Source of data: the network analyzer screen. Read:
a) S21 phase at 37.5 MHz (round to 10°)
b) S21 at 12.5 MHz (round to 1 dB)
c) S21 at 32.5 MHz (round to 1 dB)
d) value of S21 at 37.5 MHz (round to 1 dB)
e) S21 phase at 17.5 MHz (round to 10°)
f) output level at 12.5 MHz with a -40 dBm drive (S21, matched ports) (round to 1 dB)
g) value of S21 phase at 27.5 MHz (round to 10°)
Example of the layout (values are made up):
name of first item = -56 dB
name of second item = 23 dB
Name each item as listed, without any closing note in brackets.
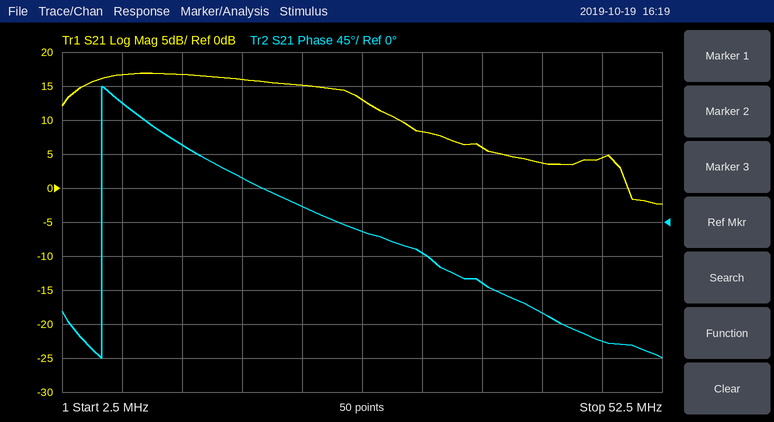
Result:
S21 phase at 37.5 MHz = -80°
S21 at 12.5 MHz = 17 dB
S21 at 32.5 MHz = 8 dB
value of S21 at 37.5 MHz = 6 dB
S21 phase at 17.5 MHz = 60°
output level at 12.5 MHz with a -40 dBm drive (S21, matched ports) = -23 dBm
value of S21 phase at 27.5 MHz = -10°
